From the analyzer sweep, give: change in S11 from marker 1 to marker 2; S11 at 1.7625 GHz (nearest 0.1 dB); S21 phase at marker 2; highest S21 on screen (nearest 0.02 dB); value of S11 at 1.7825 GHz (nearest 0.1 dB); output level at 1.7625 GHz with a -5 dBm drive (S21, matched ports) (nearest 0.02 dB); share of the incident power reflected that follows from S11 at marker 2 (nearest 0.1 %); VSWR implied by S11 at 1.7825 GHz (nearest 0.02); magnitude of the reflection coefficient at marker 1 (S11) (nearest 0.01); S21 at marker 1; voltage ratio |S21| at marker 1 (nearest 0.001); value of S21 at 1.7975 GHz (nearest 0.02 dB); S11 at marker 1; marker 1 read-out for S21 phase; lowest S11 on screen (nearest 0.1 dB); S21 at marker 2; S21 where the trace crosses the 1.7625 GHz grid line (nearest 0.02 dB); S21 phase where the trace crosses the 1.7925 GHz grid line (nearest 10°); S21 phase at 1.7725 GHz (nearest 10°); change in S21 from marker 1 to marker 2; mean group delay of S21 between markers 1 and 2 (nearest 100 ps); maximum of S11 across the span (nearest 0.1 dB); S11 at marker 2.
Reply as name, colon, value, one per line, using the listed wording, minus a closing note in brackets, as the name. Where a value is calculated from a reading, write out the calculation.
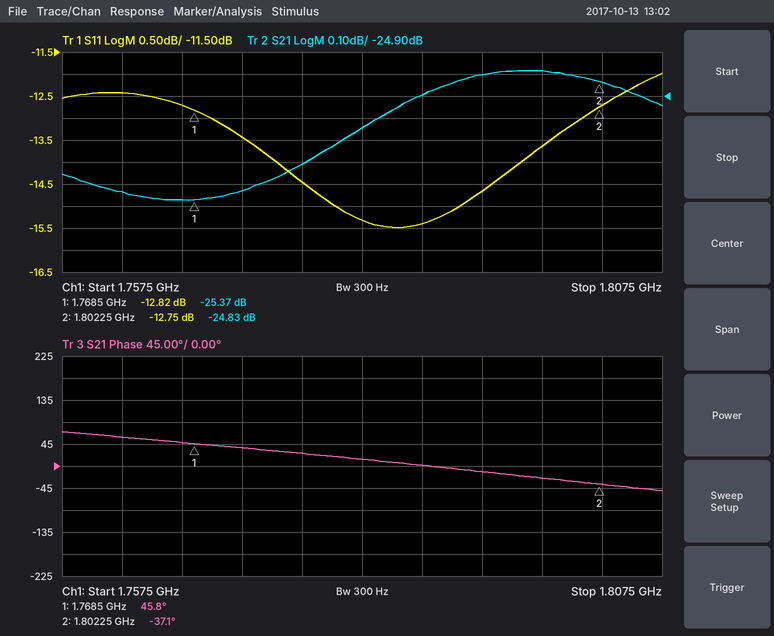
change in S11 from marker 1 to marker 2: -12.75 − (-12.82) = 0.07 dB
S11 at 1.7625 GHz: -12.4 dB
S21 phase at marker 2: -37.1°
highest S21 on screen: -24.78 dB
value of S11 at 1.7825 GHz: -15.3 dB
output level at 1.7625 GHz with a -5 dBm drive (S21, matched ports): -5 dBm + (-25.34 dB) = -30.34 dBm
share of the incident power reflected that follows from S11 at marker 2: 10^(-12.75/10) ≈ 5.3 %
VSWR implied by S11 at 1.7825 GHz: |Γ| = 10^(-15.3/20) = 0.1718; VSWR = (1 + 0.1718)/(1 − 0.1718) ≈ 1.41, so 1.42 to the nearest 0.02
magnitude of the reflection coefficient at marker 1 (S11): 10^(-12.82/20) ≈ 0.23
S21 at marker 1: -25.37 dB
voltage ratio |S21| at marker 1: 10^(-25.37/20) ≈ 0.054
value of S21 at 1.7975 GHz: -24.78 dB
S11 at marker 1: -12.82 dB
marker 1 read-out for S21 phase: 45.8°
lowest S11 on screen: -15.5 dB
S21 at marker 2: -24.83 dB
S21 where the trace crosses the 1.7625 GHz grid line: -25.34 dB
S21 phase where the trace crosses the 1.7925 GHz grid line: -10°
S21 phase at 1.7725 GHz: 40°
change in S21 from marker 1 to marker 2: -24.83 − (-25.37) = 0.54 dB
mean group delay of S21 between markers 1 and 2: −(-37.1° − (45.8°))/(360° × 33.75 MHz) ≈ 6.8 ns
maximum of S11 across the span: -12.0 dB
S11 at marker 2: -12.75 dB
